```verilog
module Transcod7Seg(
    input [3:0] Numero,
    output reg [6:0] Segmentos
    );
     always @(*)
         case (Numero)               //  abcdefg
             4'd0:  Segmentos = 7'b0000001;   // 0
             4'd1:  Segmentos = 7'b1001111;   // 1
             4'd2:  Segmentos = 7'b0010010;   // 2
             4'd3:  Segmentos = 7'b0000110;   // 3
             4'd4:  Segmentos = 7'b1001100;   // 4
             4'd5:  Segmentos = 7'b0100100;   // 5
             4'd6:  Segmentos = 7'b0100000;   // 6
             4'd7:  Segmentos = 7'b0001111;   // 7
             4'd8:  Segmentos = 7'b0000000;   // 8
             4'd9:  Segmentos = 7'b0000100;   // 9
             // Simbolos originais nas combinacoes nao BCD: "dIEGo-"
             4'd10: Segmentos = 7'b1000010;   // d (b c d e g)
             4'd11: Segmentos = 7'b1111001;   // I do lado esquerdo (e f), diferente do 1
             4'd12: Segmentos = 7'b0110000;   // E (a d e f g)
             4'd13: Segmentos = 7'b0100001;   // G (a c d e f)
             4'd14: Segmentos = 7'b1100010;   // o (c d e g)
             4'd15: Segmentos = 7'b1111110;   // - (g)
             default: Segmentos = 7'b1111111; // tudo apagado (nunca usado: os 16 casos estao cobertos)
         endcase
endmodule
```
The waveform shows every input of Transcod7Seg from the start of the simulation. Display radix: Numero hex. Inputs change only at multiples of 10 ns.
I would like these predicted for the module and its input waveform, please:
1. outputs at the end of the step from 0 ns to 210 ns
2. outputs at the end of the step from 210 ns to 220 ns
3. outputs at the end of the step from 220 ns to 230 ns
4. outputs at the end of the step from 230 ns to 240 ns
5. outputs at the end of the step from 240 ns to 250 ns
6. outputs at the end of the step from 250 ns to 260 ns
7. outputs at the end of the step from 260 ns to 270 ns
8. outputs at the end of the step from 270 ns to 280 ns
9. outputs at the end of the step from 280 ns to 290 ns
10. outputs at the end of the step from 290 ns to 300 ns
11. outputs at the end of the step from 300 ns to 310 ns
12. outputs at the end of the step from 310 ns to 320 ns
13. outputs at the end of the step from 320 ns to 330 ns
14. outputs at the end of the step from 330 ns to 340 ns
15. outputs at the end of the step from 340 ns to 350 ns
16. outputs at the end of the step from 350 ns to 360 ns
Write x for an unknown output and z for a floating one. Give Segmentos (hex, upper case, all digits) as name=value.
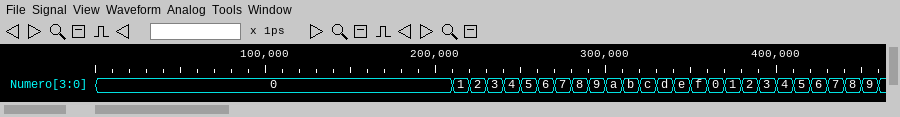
Segmentos=01
Segmentos=4F
Segmentos=12
Segmentos=06
Segmentos=4C
Segmentos=24
Segmentos=20
Segmentos=0F
Segmentos=00
Segmentos=04
Segmentos=42
Segmentos=79
Segmentos=30
Segmentos=21
Segmentos=62
Segmentos=7E
